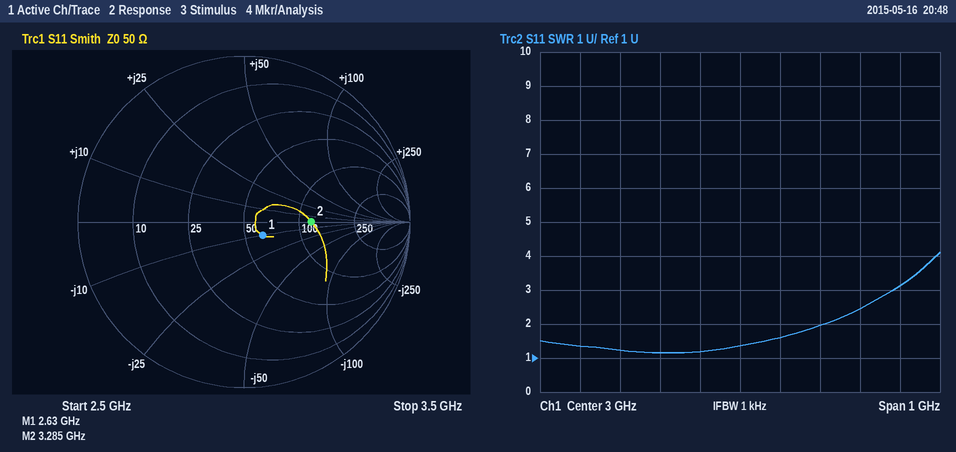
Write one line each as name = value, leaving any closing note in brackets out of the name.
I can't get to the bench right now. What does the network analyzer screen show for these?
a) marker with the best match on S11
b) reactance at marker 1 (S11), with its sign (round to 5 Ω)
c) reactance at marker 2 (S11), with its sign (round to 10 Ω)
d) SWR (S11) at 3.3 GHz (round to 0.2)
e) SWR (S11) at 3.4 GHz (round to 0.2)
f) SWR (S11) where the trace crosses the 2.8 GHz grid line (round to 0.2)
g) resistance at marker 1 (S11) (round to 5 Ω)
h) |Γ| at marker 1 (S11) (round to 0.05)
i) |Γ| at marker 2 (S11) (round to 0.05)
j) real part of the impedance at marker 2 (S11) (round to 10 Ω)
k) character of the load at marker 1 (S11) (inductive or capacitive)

marker with the best match on S11 = marker 1
reactance at marker 1 (S11), with its sign = -10 Ω
reactance at marker 2 (S11), with its sign = 0 Ω
SWR (S11) at 3.3 GHz = 2.4
SWR (S11) at 3.4 GHz = 3.2
SWR (S11) where the trace crosses the 2.8 GHz grid line = 1.2
resistance at marker 1 (S11) = 60 Ω
|Γ| at marker 1 (S11) = 0.15
|Γ| at marker 2 (S11) = 0.40
real part of the impedance at marker 2 (S11) = 120 Ω
character of the load at marker 1 (S11) = capacitive
